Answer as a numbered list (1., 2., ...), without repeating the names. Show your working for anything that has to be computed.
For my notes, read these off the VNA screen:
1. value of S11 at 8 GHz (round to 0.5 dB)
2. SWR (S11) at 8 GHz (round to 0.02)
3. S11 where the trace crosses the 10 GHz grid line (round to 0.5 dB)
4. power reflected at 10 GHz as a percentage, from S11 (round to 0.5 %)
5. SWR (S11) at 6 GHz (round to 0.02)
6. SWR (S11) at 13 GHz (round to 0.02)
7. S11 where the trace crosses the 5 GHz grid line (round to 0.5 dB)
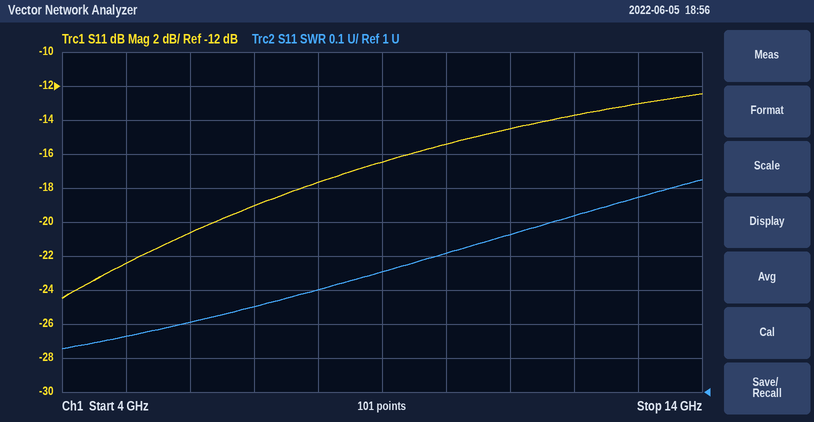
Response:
1. -17.5 dB
2. 1.30
3. -15.5 dB
4. 10^(-15.5/10) ≈ 2.82 %, so 3.0 % to the nearest 0.5 %
5. 1.20
6. 1.58
7. -22.5 dB
